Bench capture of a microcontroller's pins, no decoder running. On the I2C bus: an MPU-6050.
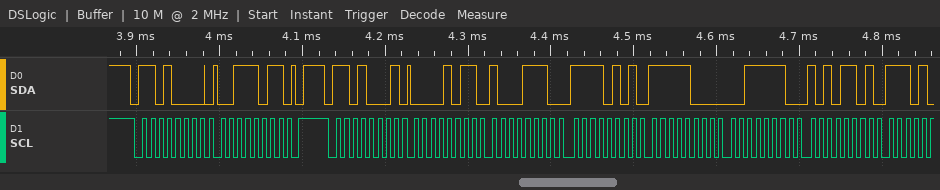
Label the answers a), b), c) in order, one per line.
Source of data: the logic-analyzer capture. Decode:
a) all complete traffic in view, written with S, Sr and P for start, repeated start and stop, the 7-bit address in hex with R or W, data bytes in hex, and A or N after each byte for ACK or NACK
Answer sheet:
a) S 68W A 3B A P S 68R A 0B A 8E A F5 A F8 A 3E A AD A
